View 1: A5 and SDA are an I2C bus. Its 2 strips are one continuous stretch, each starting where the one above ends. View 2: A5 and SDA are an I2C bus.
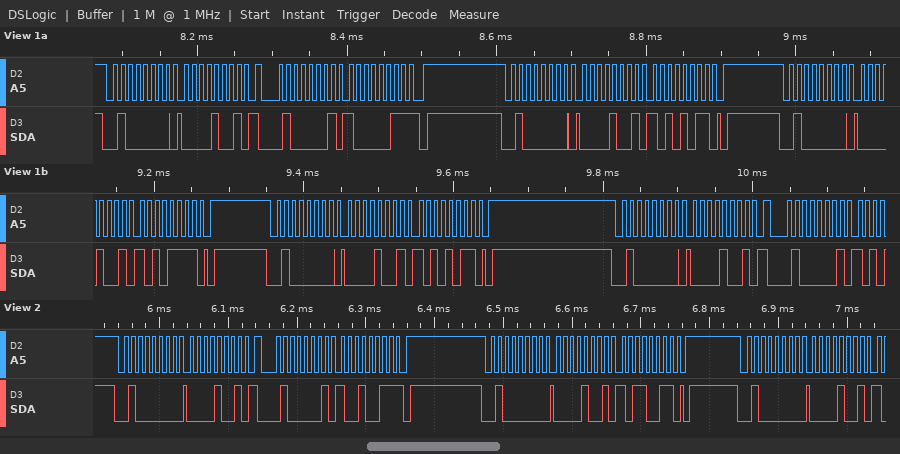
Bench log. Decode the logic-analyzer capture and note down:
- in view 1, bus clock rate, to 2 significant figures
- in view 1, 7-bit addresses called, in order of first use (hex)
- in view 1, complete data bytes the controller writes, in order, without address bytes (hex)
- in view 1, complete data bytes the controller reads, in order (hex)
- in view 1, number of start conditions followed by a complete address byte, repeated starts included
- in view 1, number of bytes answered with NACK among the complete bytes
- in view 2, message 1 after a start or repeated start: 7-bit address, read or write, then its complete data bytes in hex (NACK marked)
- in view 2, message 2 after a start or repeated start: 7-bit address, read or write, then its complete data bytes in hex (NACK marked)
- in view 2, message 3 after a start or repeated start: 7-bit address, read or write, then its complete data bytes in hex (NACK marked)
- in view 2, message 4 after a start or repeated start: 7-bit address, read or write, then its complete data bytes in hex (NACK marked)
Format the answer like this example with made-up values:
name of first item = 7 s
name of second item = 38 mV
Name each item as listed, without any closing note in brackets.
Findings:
in view 1, bus clock rate, to 2 significant figures = 100 kHz
in view 1, 7-bit addresses called, in order of first use = 0x20
in view 1, complete data bytes the controller writes, in order, without address bytes = 09 09 AB 09 AF 09 AB 09
in view 1, complete data bytes the controller reads, in order = 83
in view 1, number of start conditions followed by a complete address byte, repeated starts included = 7
in view 1, number of bytes answered with NACK among the complete bytes = 1
in view 2, message 1 after a start or repeated start: 7-bit address, read or write, then its complete data bytes in hex = 0x20 write: 09
in view 2, message 2 after a start or repeated start: 7-bit address, read or write, then its complete data bytes in hex = 0x20 read: 93 NACK
in view 2, message 3 after a start or repeated start: 7-bit address, read or write, then its complete data bytes in hex = 0x20 write: 09 B3
in view 2, message 4 after a start or repeated start: 7-bit address, read or write, then its complete data bytes in hex = 0x20 write: 09
